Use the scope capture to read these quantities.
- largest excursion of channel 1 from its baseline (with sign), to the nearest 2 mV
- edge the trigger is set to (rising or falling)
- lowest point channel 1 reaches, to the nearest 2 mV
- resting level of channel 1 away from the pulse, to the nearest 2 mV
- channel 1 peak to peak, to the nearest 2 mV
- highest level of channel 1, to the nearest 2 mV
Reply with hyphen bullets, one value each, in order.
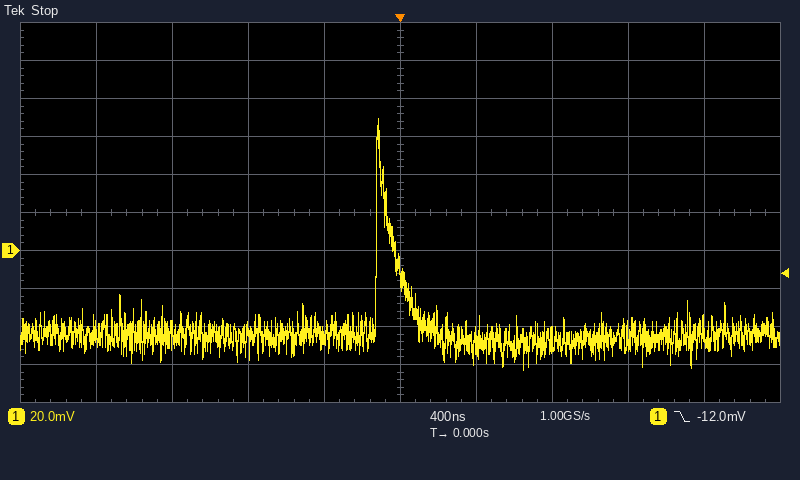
- +114 mV
- falling
- -62 mV
- -44 mV
- 132 mV
- 70 mV
